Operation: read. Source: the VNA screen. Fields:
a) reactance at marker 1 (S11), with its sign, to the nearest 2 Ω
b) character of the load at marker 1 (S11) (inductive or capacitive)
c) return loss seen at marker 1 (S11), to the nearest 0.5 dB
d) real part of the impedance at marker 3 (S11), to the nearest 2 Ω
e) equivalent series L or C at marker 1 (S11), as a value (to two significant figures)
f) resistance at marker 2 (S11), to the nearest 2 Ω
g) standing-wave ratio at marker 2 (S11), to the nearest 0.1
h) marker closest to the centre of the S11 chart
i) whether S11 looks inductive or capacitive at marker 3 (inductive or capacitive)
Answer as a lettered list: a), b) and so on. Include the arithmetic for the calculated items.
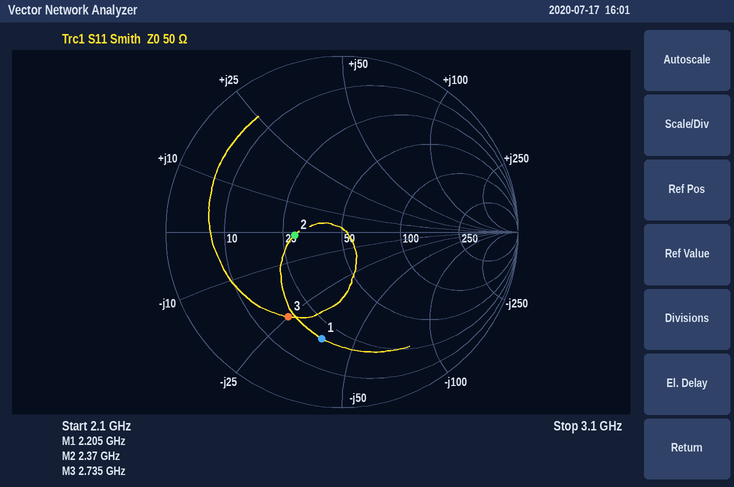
a) -38 Ω
b) capacitive
c) 4.0 dB
d) 18 Ω
e) C = 1/(2π × 2.205 GHz × 38 Ω) ≈ 1.9 pF
f) 28 Ω
g) 1.7
h) marker 2
i) capacitive
